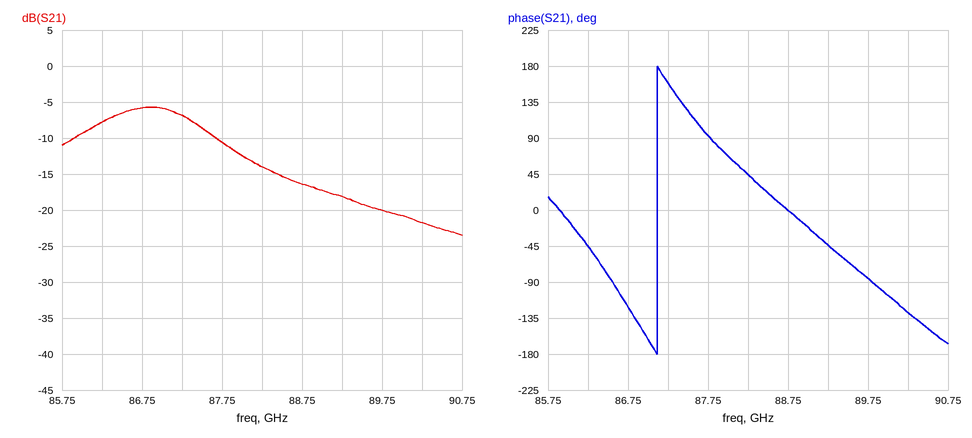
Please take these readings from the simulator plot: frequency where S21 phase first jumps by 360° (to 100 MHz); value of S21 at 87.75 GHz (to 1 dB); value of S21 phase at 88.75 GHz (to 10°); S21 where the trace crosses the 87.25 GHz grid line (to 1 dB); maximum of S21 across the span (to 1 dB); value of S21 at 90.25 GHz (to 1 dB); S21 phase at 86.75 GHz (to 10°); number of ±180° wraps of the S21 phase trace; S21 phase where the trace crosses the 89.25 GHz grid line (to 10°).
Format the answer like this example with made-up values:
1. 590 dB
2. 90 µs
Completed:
1. 87.1 GHz
2. -11 dB
3. 0°
4. -7 dB
5. -6 dB
6. -22 dB
7. -120°
8. 1
9. -40°
